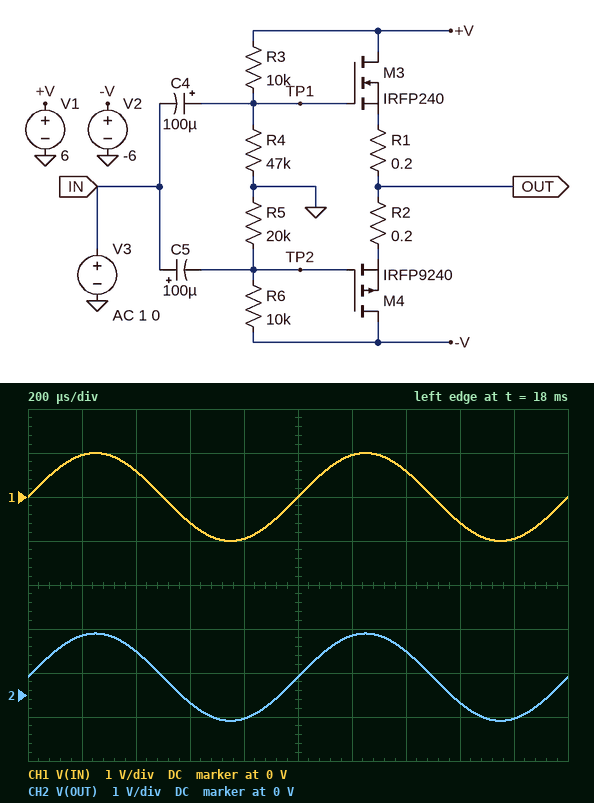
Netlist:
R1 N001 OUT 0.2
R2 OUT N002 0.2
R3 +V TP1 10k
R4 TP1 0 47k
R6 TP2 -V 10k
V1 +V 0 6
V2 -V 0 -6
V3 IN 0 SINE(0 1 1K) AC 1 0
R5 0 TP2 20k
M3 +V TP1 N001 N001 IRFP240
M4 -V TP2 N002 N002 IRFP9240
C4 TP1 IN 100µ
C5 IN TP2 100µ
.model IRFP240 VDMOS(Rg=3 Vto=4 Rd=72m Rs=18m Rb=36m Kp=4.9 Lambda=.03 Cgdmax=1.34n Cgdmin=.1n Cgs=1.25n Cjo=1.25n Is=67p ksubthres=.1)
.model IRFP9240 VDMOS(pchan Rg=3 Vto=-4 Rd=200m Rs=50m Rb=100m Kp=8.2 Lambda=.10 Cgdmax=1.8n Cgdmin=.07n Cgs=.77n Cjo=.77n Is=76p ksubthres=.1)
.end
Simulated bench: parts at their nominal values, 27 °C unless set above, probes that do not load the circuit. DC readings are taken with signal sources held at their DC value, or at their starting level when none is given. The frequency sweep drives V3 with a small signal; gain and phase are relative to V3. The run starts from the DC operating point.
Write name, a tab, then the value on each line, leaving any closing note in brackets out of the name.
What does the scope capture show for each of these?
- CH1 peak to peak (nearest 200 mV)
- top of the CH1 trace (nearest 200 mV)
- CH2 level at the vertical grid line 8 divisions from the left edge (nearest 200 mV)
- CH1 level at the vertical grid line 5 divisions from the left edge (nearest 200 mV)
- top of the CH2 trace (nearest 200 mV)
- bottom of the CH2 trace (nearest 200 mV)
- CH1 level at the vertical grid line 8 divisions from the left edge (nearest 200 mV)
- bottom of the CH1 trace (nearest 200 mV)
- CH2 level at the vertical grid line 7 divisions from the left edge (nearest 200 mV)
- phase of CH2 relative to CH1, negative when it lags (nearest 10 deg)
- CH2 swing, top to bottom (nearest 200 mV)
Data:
CH1 peak to peak	2.0 V
top of the CH1 trace	1.0 V
CH2 level at the vertical grid line 8 divisions from the left edge	-200 mV
CH1 level at the vertical grid line 5 divisions from the left edge	0 V
top of the CH2 trace	1.4 V
bottom of the CH2 trace	-600 mV
CH1 level at the vertical grid line 8 divisions from the left edge	-600 mV
bottom of the CH1 trace	-1.0 V
CH2 level at the vertical grid line 7 divisions from the left edge	1.0 V
phase of CH2 relative to CH1, negative when it lags	0 deg
CH2 swing, top to bottom	2.0 V
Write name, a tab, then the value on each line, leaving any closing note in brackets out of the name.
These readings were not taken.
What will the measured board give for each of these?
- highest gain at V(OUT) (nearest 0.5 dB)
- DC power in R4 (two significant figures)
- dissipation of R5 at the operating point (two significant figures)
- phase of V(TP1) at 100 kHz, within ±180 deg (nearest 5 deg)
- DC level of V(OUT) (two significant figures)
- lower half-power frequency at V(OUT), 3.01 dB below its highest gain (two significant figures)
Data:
highest gain at V(OUT)	0 dB
DC power in R4	520 µW
dissipation of R5 at the operating point	800 µW
phase of V(TP1) at 100 kHz, within ±180 deg	0 deg
DC level of V(OUT)	410 mV
lower half-power frequency at V(OUT), 3.01 dB below its highest gain	220 mHz
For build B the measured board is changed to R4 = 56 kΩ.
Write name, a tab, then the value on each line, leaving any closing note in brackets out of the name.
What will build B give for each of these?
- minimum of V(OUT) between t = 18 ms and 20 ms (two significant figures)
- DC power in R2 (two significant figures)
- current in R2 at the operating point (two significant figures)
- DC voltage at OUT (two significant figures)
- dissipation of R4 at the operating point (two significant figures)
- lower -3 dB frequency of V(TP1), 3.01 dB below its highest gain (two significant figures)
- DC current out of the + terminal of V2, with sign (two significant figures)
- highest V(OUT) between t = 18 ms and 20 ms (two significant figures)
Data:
minimum of V(OUT) between t = 18 ms and 20 ms	-520 mV
DC power in R2	85 mW
current in R2 at the operating point	650 mA
DC voltage at OUT	470 mV
dissipation of R4 at the operating point	460 µW
lower -3 dB frequency of V(TP1), 3.01 dB below its highest gain	190 mHz
DC current out of the + terminal of V2, with sign	-650 mA
highest V(OUT) between t = 18 ms and 20 ms	1.5 V
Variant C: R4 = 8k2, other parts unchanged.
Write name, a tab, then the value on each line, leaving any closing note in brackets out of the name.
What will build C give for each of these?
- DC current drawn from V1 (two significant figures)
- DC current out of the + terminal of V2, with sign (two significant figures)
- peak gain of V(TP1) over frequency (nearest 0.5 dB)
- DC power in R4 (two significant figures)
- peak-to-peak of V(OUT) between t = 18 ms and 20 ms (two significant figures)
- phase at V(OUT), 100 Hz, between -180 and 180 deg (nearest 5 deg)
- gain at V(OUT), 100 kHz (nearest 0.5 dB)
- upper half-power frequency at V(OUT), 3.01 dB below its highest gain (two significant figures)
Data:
DC current drawn from V1	330 µA
DC current out of the + terminal of V2, with sign	-200 µA
peak gain of V(TP1) over frequency	0 dB
DC power in R4	890 µW
peak-to-peak of V(OUT) between t = 18 ms and 20 ms	1.7 V
phase at V(OUT), 100 Hz, between -180 and 180 deg	-5 deg
gain at V(OUT), 100 kHz	-2.5 dB
upper half-power frequency at V(OUT), 3.01 dB below its highest gain	32 MHz
